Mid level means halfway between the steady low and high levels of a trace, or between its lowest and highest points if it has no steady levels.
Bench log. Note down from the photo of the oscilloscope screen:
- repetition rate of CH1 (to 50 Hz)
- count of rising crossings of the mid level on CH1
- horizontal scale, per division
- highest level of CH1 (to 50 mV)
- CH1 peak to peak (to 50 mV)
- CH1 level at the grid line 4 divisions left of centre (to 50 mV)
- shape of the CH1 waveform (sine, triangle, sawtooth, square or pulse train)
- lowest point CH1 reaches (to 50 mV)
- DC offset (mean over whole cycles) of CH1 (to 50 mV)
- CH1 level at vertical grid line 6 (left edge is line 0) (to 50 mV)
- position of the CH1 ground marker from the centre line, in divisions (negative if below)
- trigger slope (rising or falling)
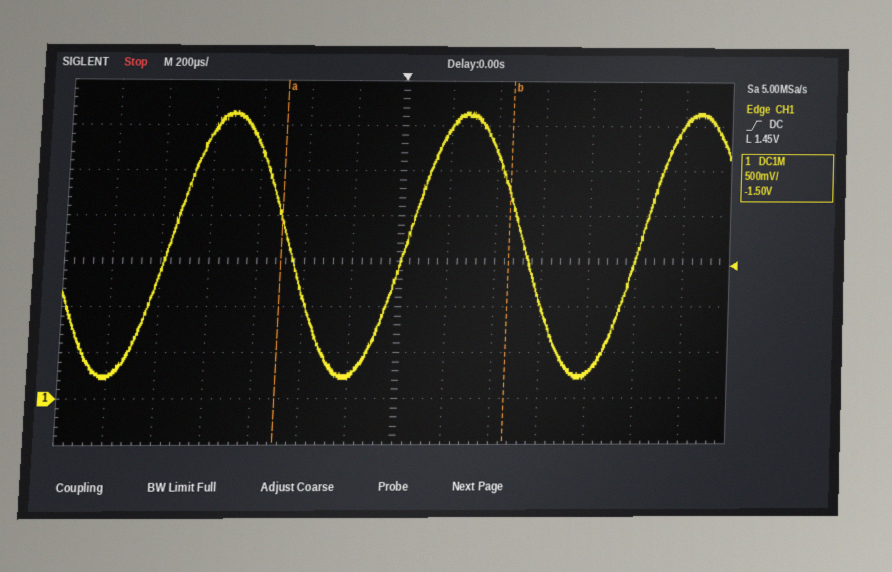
1.00 kHz
3
200 µs
3.15 V
2.95 V
2.95 V
sine
200 mV
1.70 V
250 mV
-3.0 div
rising
